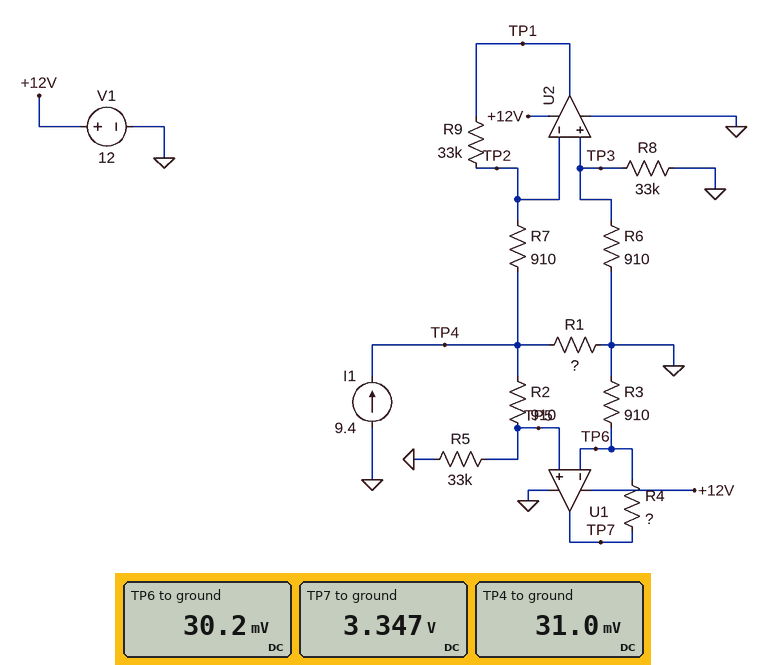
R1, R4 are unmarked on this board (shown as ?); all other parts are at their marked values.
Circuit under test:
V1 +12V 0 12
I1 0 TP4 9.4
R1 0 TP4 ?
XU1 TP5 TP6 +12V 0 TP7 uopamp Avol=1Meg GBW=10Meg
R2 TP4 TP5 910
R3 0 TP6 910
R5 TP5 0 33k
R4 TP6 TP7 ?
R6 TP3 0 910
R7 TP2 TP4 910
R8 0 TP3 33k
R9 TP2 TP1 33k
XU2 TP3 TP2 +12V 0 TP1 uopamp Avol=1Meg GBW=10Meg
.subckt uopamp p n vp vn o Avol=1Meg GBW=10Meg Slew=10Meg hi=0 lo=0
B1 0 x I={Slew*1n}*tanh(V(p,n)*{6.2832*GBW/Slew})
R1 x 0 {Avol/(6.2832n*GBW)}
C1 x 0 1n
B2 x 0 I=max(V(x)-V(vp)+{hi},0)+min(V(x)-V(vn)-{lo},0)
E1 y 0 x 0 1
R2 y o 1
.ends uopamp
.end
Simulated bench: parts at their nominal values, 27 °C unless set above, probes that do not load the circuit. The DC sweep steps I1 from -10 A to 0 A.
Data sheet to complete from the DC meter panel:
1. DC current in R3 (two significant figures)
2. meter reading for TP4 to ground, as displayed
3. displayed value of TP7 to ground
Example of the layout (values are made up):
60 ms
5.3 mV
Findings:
33 µA
31.0 mV
3.347 V
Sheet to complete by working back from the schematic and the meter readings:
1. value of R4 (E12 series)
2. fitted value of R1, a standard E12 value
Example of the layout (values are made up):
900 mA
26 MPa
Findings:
100 kΩ
3.3 mΩ
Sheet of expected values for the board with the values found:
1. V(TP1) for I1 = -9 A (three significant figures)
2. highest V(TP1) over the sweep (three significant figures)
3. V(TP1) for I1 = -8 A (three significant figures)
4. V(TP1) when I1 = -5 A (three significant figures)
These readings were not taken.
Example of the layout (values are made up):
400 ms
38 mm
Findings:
1.08 V
1.20 V
957 mV
598 mV
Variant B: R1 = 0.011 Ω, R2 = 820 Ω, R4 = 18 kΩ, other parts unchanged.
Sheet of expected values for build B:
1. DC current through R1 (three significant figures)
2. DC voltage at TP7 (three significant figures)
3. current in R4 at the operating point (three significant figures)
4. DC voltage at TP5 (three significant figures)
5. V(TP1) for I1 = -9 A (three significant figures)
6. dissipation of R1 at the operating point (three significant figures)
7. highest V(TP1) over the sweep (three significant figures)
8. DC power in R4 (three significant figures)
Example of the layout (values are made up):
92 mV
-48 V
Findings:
9.40 A
2.10 V
111 µA
101 mV
3.59 V
972 mW
3.99 V
221 µW
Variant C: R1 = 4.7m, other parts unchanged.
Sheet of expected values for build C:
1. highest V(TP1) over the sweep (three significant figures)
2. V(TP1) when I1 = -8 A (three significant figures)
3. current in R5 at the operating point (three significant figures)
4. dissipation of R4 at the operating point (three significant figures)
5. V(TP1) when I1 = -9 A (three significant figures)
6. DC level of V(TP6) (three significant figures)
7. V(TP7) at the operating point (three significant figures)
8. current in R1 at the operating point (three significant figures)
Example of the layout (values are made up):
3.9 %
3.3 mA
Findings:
1.70 V
1.36 V
1.30 µA
223 µW
1.53 V
43.0 mV
4.77 V
9.40 A
